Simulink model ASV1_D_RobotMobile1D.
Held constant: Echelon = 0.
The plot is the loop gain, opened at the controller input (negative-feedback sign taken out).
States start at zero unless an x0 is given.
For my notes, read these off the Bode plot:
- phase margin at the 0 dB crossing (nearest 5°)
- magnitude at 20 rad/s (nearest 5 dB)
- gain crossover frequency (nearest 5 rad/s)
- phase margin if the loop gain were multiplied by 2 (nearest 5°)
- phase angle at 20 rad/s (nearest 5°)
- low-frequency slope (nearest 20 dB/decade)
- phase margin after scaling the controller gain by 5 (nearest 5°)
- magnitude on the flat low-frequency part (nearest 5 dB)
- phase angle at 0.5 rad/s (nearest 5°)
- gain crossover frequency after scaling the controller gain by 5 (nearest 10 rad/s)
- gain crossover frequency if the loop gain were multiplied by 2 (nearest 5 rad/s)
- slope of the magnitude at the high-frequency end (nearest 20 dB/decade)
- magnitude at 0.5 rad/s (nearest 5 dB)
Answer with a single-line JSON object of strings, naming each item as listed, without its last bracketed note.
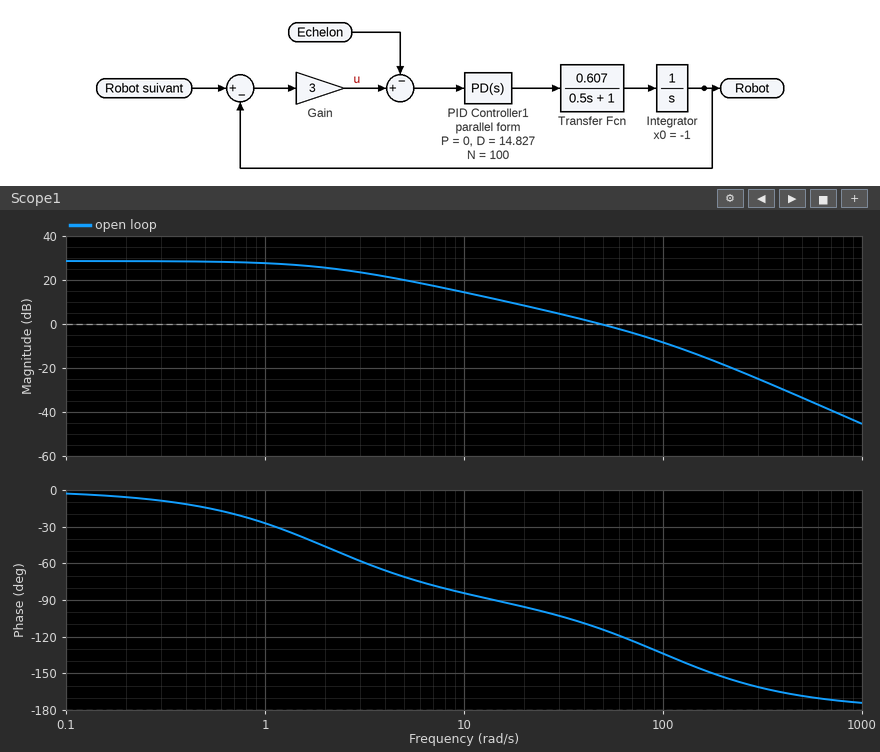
{"phase margin at the 0 dB crossing": "65°", "magnitude at 20 rad/s": "10 dB", "gain crossover frequency": "50 rad/s", "phase margin if the loop gain were multiplied by 2": "50°", "phase angle at 20 rad/s": "-95°", "low-frequency slope": "0 dB/decade", "phase margin after scaling the controller gain by 5": "35°", "magnitude on the flat low-frequency part": "30 dB", "phase angle at 0.5 rad/s": "-15°", "gain crossover frequency after scaling the controller gain by 5": "150 rad/s", "gain crossover frequency if the loop gain were multiplied by 2": "85 rad/s", "slope of the magnitude at the high-frequency end": "-40 dB/decade", "magnitude at 0.5 rad/s": "30 dB"}
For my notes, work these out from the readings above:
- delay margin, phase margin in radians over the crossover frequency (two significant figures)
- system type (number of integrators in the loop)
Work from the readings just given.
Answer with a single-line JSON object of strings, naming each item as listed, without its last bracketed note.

{"delay margin, phase margin in radians over the crossover frequency": "0.023 s", "system type": "0"}
